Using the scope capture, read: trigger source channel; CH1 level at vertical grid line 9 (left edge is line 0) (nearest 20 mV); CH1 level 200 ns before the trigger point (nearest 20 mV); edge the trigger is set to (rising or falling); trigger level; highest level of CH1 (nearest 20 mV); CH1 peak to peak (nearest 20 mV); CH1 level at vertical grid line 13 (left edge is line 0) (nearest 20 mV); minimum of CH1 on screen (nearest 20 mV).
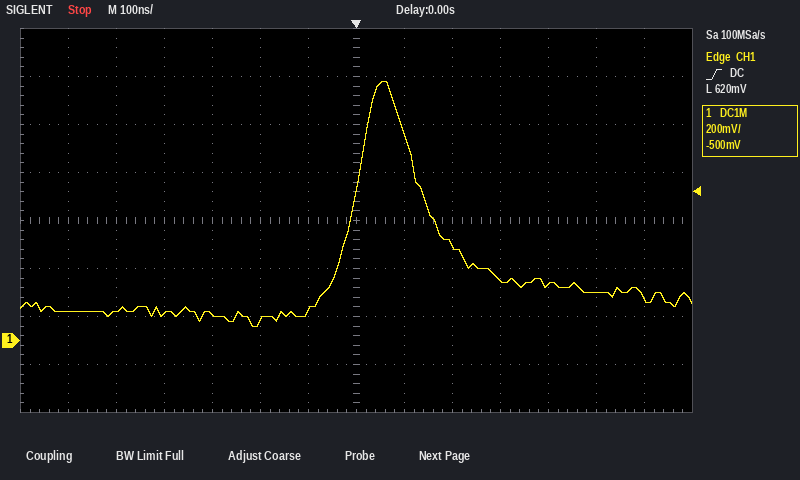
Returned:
CH1
400 mV
80 mV
rising
620 mV
1.08 V
1.02 V
180 mV
60 mV
